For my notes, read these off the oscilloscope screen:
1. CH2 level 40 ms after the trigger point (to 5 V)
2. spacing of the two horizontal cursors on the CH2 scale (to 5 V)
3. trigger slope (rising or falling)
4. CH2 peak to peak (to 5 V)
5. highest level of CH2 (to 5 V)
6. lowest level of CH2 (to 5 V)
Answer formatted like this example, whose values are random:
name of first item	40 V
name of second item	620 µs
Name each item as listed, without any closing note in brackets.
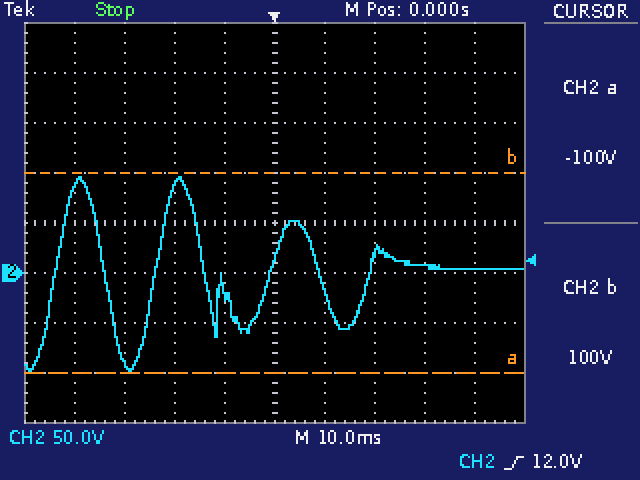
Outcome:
CH2 level 40 ms after the trigger point	5 V
spacing of the two horizontal cursors on the CH2 scale	200 V
trigger slope	rising
CH2 peak to peak	195 V
highest level of CH2	95 V
lowest level of CH2	-100 V
